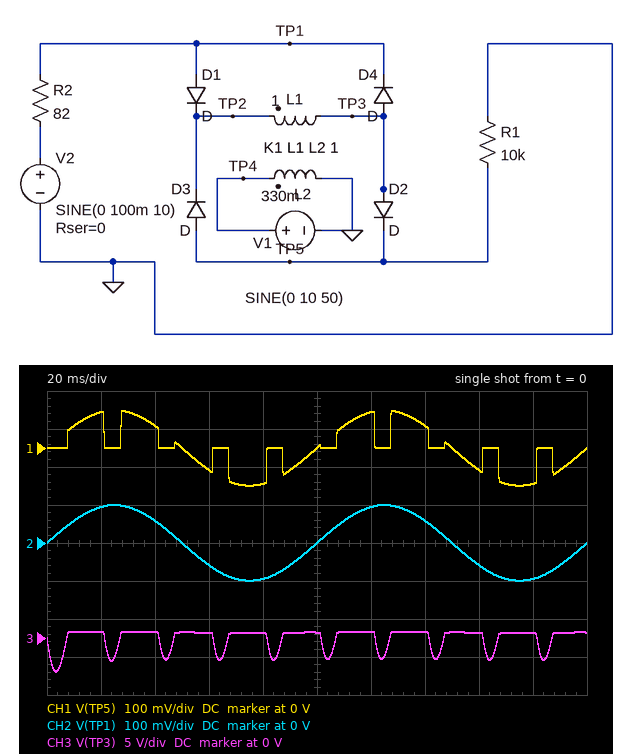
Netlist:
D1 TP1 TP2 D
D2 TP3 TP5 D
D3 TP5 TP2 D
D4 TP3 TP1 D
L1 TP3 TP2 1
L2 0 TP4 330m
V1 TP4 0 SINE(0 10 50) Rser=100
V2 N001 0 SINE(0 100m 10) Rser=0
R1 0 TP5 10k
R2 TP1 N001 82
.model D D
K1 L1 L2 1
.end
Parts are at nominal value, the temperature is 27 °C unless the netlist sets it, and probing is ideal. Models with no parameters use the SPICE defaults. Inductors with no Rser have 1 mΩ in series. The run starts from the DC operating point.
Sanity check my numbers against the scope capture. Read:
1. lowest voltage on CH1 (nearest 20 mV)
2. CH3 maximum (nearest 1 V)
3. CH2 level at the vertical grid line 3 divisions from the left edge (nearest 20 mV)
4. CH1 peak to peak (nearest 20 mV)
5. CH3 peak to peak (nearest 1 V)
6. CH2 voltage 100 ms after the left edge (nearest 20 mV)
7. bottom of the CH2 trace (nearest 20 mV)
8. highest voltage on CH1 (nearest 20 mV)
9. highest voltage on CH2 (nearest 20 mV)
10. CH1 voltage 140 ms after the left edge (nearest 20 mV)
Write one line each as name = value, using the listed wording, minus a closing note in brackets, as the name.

lowest voltage on CH1 = -100 mV
CH3 maximum = 1 V
CH2 level at the vertical grid line 3 divisions from the left edge = -60 mV
CH1 peak to peak = 200 mV
CH3 peak to peak = 5 V
CH2 voltage 100 ms after the left edge = 0 V
bottom of the CH2 trace = -100 mV
highest voltage on CH1 = 100 mV
highest voltage on CH2 = 100 mV
CH1 voltage 140 ms after the left edge = 60 mV
